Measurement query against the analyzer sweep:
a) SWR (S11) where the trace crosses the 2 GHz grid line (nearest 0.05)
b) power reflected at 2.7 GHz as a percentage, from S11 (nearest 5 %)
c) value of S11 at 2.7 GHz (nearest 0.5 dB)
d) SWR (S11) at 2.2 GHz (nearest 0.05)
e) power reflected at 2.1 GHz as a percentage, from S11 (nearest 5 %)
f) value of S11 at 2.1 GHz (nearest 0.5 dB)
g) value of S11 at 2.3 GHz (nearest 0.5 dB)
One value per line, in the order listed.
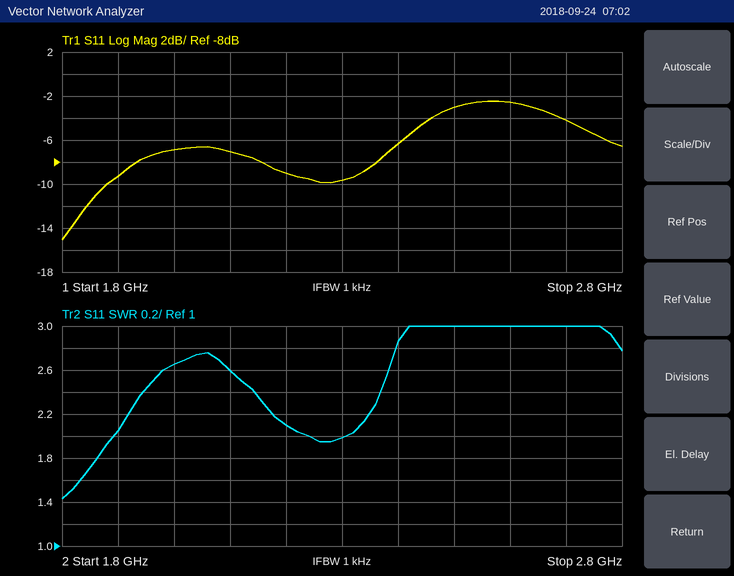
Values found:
2.65
40 %
-4.0 dB
2.10
20 %
-7.0 dB
-9.5 dB
